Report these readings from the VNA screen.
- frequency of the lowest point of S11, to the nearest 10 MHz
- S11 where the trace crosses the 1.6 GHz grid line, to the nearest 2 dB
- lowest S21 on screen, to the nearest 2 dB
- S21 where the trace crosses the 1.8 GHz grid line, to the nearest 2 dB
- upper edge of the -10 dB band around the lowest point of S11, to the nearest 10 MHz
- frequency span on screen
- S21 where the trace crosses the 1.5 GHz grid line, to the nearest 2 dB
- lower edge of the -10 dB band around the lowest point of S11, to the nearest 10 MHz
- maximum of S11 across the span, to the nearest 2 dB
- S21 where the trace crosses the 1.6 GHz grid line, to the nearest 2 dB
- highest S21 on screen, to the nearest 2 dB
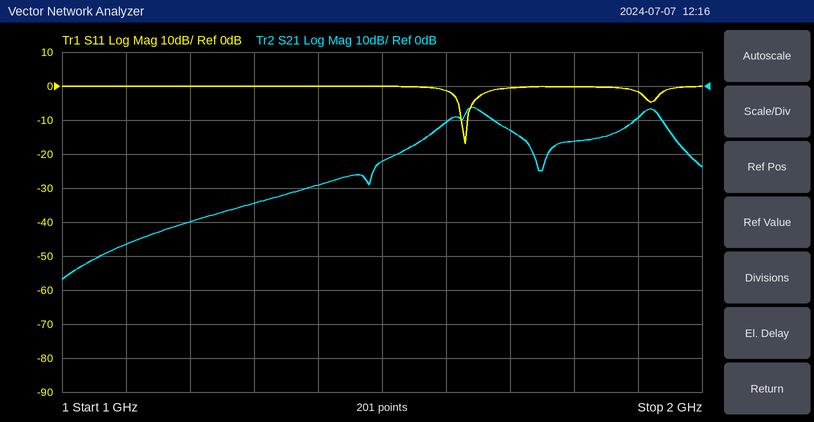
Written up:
1.63 GHz
-2 dB
-56 dB
-16 dB
1.63 GHz
1 GHz
-22 dB
1.62 GHz
0 dB
-10 dB
-6 dB
